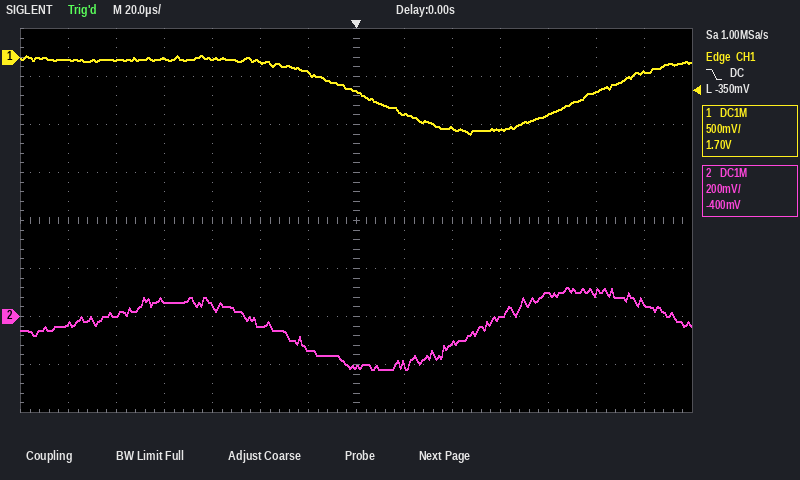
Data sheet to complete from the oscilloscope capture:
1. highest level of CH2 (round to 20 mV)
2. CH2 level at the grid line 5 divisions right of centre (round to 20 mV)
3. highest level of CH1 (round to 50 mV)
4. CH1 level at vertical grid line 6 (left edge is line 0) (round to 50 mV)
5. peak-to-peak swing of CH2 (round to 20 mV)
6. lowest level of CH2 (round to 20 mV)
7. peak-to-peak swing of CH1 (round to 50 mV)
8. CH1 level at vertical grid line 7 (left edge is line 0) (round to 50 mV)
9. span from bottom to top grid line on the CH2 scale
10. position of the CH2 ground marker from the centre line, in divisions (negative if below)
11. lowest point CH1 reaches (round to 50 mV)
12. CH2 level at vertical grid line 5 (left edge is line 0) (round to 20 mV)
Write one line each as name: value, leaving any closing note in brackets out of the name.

highest level of CH2: 120 mV
CH2 level at the grid line 5 divisions right of centre: 100 mV
highest level of CH1: 0 mV
CH1 level at vertical grid line 6 (left edge is line 0): -150 mV
peak-to-peak swing of CH2: 340 mV
lowest level of CH2: -220 mV
peak-to-peak swing of CH1: 800 mV
CH1 level at vertical grid line 7 (left edge is line 0): -350 mV
span from bottom to top grid line on the CH2 scale: 1.6 V
position of the CH2 ground marker from the centre line, in divisions: -2.0 div
lowest point CH1 reaches: -800 mV
CH2 level at vertical grid line 5 (left edge is line 0): -40 mV
